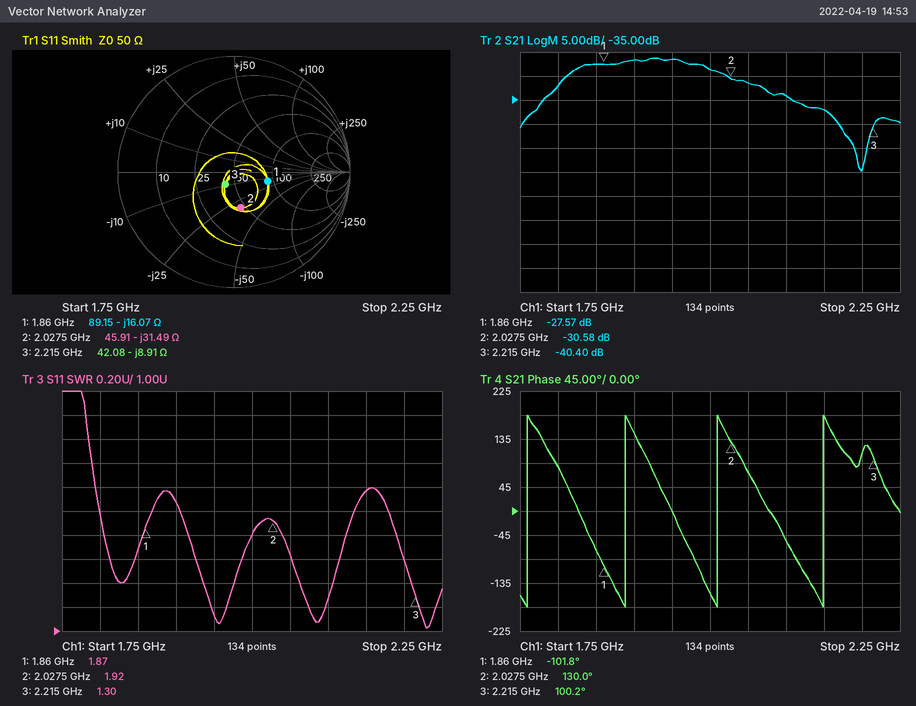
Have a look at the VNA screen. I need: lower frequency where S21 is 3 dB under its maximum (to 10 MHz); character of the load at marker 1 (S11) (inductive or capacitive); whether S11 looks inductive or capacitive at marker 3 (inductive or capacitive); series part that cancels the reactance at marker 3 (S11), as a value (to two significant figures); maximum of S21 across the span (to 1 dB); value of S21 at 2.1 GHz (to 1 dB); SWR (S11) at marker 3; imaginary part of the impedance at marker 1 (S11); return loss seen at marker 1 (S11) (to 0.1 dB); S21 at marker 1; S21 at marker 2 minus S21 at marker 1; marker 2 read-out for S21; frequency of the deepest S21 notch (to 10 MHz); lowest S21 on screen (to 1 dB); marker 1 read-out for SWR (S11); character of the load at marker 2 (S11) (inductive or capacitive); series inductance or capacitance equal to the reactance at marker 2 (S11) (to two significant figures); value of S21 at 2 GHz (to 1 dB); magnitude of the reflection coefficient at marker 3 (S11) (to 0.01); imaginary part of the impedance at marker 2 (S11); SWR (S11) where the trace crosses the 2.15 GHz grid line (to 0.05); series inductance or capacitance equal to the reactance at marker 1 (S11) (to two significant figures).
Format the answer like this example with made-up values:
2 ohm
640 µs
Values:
1.82 GHz
capacitive
capacitive
640 pH
-26 dB
-34 dB
1.30
-16.07 Ω
10.4 dB
-27.57 dB
-3.01 dB
-30.58 dB
2.20 GHz
-50 dB
1.87
capacitive
2.5 pF
-29 dB
0.13
-31.49 Ω
2.15
5.3 pF
